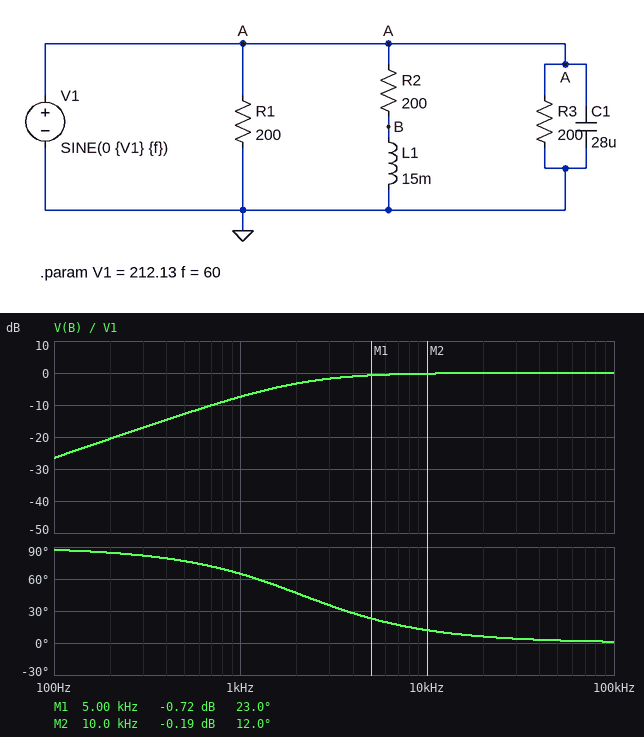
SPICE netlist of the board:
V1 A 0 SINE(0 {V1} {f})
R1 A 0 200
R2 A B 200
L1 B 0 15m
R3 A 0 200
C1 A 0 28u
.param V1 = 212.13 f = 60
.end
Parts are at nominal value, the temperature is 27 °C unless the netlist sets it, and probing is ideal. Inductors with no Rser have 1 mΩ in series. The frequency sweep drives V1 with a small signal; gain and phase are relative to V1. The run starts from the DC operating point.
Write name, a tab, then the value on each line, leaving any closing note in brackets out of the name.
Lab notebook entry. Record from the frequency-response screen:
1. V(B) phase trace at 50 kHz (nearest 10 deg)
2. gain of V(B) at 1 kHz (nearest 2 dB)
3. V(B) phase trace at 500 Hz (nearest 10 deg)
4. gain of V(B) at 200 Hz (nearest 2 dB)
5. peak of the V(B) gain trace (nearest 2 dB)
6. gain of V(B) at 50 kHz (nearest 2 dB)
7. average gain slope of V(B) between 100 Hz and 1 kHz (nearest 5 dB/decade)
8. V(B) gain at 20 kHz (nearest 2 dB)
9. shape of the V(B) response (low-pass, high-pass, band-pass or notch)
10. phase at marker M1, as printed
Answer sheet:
V(B) phase trace at 50 kHz	0 deg
gain of V(B) at 1 kHz	-8 dB
V(B) phase trace at 500 Hz	80 deg
gain of V(B) at 200 Hz	-20 dB
peak of the V(B) gain trace	0 dB
gain of V(B) at 50 kHz	0 dB
average gain slope of V(B) between 100 Hz and 1 kHz	20 dB/decade
V(B) gain at 20 kHz	0 dB
shape of the V(B) response	high-pass
phase at marker M1, as printed	23.0 deg
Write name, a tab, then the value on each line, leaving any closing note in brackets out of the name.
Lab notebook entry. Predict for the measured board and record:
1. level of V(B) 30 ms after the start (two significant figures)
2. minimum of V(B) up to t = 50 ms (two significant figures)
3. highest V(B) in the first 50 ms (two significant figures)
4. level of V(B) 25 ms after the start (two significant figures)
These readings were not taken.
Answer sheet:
level of V(B) 30 ms after the start	1.7 V
minimum of V(B) up to t = 50 ms	-6.0 V
highest V(B) in the first 50 ms	6.0 V
level of V(B) 25 ms after the start	-6.0 V
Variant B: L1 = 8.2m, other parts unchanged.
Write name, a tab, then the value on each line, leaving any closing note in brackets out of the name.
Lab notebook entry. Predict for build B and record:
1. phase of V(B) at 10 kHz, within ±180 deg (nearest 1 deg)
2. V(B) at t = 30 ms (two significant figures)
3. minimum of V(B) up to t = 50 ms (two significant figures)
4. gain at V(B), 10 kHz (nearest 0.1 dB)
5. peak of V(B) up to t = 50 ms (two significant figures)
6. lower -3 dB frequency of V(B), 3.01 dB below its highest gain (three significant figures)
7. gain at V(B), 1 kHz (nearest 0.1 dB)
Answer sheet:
phase of V(B) at 10 kHz, within ±180 deg	21 deg
V(B) at t = 30 ms	960 mV
minimum of V(B) up to t = 50 ms	-3.3 V
gain at V(B), 10 kHz	-0.6 dB
peak of V(B) up to t = 50 ms	3.3 V
lower -3 dB frequency of V(B), 3.01 dB below its highest gain	3.88 kHz
gain at V(B), 1 kHz	-12.1 dB
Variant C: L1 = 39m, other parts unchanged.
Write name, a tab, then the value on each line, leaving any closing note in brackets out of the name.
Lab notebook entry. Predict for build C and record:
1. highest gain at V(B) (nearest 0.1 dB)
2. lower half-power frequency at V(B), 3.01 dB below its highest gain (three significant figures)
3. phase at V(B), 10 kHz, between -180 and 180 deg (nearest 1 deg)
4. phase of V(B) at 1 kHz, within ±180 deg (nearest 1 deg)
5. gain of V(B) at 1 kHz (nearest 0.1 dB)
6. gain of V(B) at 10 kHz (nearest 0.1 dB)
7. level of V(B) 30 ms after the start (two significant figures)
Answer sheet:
highest gain at V(B)	0 dB
lower half-power frequency at V(B), 3.01 dB below its highest gain	816 Hz
phase at V(B), 10 kHz, between -180 and 180 deg	5 deg
phase of V(B) at 1 kHz, within ±180 deg	39 deg
gain of V(B) at 1 kHz	-2.2 dB
gain of V(B) at 10 kHz	0 dB
level of V(B) 30 ms after the start	3.7 V
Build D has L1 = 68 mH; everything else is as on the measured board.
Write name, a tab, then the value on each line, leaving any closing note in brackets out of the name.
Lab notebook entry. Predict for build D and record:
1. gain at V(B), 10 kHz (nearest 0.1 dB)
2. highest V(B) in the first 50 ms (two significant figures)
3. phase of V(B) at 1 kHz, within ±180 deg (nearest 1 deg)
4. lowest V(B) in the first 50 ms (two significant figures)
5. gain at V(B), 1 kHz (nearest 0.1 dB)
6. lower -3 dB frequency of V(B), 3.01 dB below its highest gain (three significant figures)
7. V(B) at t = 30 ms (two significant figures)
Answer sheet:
gain at V(B), 10 kHz	0 dB
highest V(B) in the first 50 ms	27 V
phase of V(B) at 1 kHz, within ±180 deg	25 deg
lowest V(B) in the first 50 ms	-27 V
gain at V(B), 1 kHz	-0.9 dB
lower -3 dB frequency of V(B), 3.01 dB below its highest gain	468 Hz
V(B) at t = 30 ms	5.0 V
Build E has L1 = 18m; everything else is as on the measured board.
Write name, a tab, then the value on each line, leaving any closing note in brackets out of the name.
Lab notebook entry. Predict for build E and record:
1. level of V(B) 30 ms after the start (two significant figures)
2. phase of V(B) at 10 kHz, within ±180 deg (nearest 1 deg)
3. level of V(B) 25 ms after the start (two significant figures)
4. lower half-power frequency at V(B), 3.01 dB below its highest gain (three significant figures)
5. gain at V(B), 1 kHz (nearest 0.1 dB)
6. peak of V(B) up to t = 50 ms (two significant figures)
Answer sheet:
level of V(B) 30 ms after the start	2.0 V
phase of V(B) at 10 kHz, within ±180 deg	10 deg
level of V(B) 25 ms after the start	-7.2 V
lower half-power frequency at V(B), 3.01 dB below its highest gain	1.77 kHz
gain at V(B), 1 kHz	-6.2 dB
peak of V(B) up to t = 50 ms	7.2 V
